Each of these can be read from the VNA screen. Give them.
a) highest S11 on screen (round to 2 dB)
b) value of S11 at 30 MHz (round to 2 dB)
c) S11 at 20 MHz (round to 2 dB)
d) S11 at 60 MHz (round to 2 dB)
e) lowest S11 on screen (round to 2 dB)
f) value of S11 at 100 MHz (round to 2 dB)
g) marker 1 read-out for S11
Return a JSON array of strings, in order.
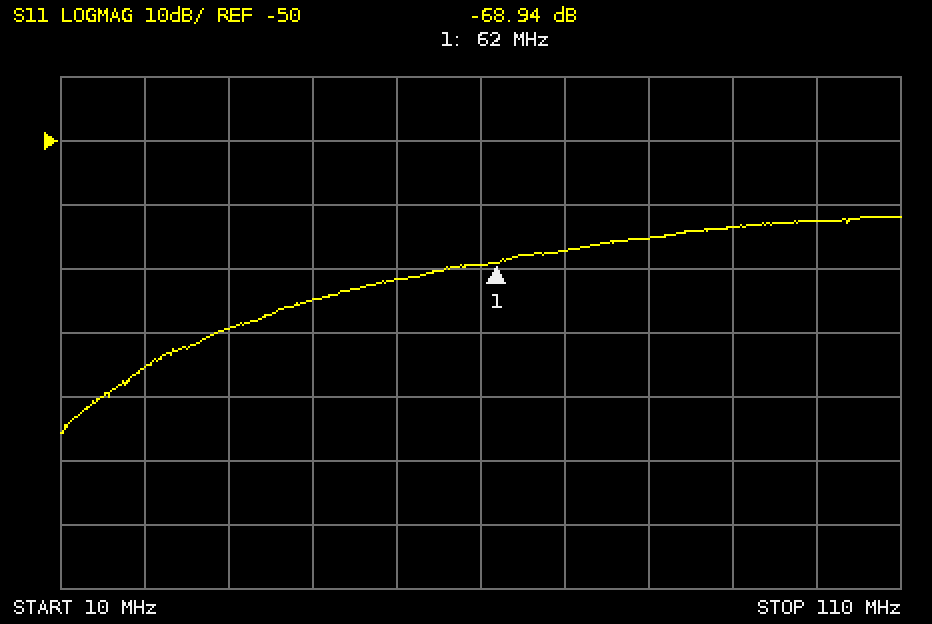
["-62 dB", "-80 dB", "-86 dB", "-70 dB", "-96 dB", "-62 dB", "-68.94 dB"]
